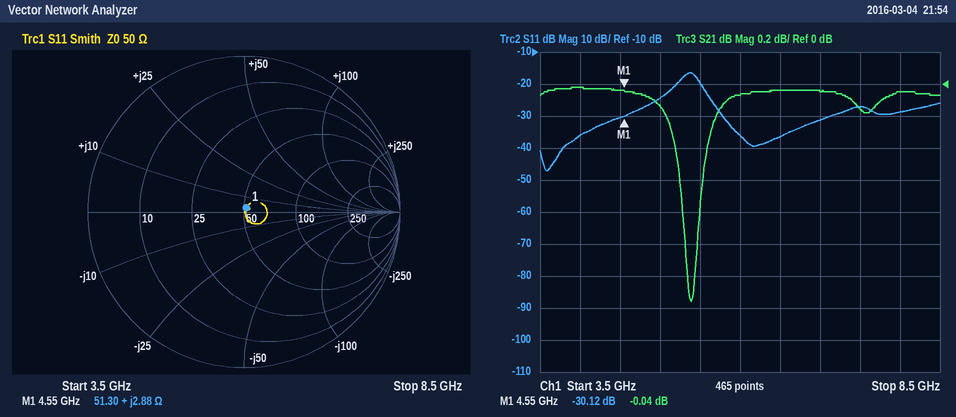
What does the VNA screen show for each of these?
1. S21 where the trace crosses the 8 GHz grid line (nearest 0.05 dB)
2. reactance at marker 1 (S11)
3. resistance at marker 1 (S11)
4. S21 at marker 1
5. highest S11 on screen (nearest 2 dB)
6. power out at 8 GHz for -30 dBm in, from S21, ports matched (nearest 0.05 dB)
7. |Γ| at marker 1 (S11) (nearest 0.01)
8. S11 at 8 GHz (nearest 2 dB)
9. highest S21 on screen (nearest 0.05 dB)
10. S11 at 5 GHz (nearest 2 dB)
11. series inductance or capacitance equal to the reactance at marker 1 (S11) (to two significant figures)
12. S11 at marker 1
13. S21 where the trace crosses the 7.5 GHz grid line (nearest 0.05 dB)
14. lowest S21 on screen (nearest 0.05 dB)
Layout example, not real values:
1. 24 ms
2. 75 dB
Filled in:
1. -0.05 dB
2. +2.88 Ω
3. 51.30 Ω
4. -0.04 dB
5. -16 dB
6. -30.05 dBm
7. 0.03
8. -28 dB
9. 0.00 dB
10. -24 dB
11. 100 pH
12. -30.12 dB
13. -0.15 dB
14. -1.35 dB
